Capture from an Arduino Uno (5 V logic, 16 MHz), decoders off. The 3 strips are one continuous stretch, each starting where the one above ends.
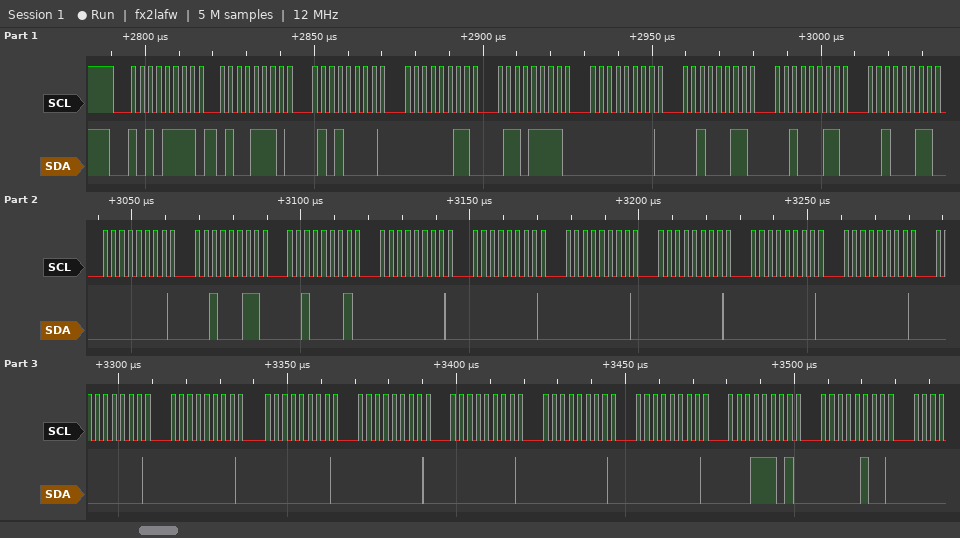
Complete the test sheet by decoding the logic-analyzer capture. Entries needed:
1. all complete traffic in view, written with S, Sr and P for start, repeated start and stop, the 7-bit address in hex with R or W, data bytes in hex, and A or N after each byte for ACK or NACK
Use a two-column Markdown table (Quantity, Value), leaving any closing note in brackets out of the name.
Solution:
| Quantity | Value |
|---|---|
| all complete traffic in view, written with S, Sr and P for start, repeated start and stop, the 7-bit address in hex with R or W, data bytes in hex, and A or N after each byte for ACK or NACK | S 57R A 4E A 50 A 03 A 6F A 00 A 23 A 23 A 23 A 00 A 23 A 21 A 00 A 00 A 00 A 00 A 00 A 00 A 00 A 00 A 00 A 00 A 00 A 00 A 00 A 1D A 04 A |
